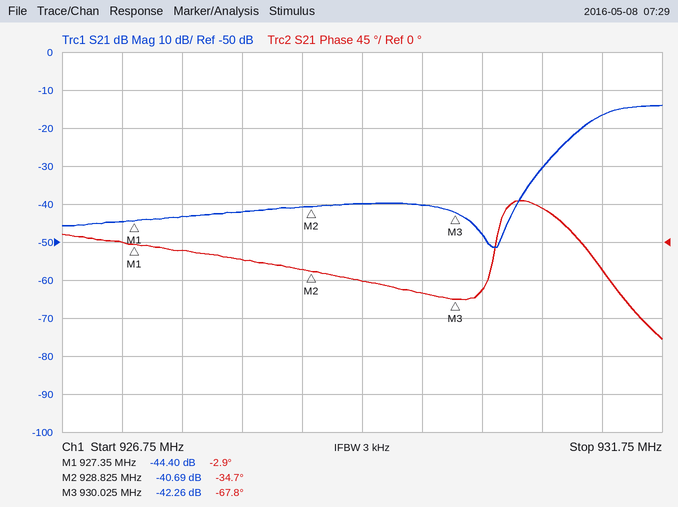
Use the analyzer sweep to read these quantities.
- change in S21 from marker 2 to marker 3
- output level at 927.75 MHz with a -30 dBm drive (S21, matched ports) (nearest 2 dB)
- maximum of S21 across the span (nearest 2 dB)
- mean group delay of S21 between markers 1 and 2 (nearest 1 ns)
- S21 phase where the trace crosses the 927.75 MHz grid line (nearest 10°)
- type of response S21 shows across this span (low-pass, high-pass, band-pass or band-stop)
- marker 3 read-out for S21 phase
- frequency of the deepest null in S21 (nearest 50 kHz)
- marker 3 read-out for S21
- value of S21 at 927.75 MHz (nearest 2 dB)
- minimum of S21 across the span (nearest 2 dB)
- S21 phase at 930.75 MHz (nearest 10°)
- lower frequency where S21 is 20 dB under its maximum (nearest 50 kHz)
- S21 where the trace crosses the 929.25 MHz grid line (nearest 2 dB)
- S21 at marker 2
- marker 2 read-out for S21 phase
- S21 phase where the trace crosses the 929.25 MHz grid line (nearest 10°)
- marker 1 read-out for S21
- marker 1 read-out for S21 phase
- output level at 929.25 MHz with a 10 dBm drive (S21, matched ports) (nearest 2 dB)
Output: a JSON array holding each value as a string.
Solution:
["-1.57 dB", "-74 dBm", "-14 dB", "60 ns", "-10°", "high-pass", "-67.8°", "930.35 MHz", "-42.26 dB", "-44 dB", "-52 dB", "40°", "930.65 MHz", "-40 dB", "-40.69 dB", "-34.7°", "-50°", "-44.40 dB", "-2.9°", "-30 dBm"]
